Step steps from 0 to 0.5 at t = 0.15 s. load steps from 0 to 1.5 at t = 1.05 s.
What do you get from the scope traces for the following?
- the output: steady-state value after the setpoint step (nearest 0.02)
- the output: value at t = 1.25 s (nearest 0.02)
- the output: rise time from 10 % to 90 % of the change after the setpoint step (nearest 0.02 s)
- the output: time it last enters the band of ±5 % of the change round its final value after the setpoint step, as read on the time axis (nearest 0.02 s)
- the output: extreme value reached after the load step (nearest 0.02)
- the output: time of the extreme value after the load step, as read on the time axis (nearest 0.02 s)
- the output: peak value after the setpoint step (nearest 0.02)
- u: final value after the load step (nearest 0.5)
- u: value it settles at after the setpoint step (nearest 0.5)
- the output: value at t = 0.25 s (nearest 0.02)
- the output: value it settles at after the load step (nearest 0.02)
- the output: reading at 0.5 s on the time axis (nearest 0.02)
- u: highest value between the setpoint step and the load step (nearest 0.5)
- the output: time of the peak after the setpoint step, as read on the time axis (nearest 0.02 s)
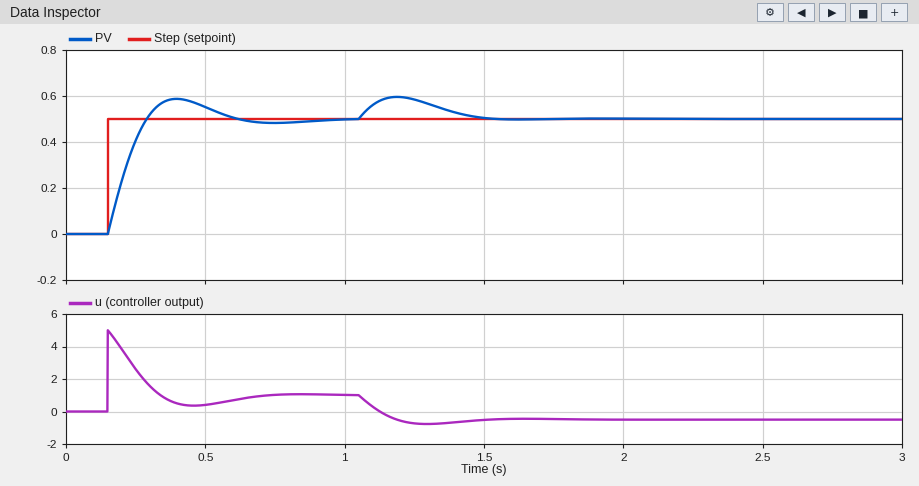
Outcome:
0.50
0.58
0.10 s
0.56 s
0.60
1.18 s
0.58
-0.5
1.0
0.40
0.50
0.56
5.0
0.40 s
